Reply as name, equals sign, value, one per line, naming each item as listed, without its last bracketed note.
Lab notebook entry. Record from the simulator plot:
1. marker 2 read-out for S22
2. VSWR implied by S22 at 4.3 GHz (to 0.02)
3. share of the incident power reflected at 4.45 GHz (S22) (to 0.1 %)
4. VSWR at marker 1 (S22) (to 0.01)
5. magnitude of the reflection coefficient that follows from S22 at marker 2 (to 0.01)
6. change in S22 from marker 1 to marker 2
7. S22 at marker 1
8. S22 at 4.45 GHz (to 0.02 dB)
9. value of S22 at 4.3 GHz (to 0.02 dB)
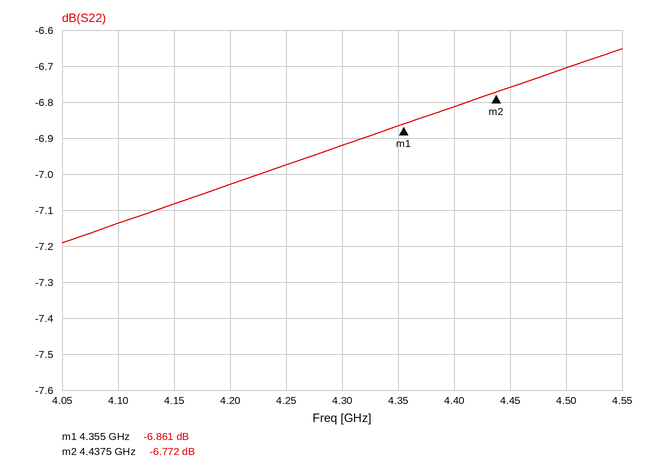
marker 2 read-out for S22 = -6.772 dB
VSWR implied by S22 at 4.3 GHz = 2.64
share of the incident power reflected at 4.45 GHz (S22) = 21.1 %
VSWR at marker 1 (S22) = 2.66
magnitude of the reflection coefficient that follows from S22 at marker 2 = 0.46
change in S22 from marker 1 to marker 2 = 0.089 dB
S22 at marker 1 = -6.861 dB
S22 at 4.45 GHz = -6.76 dB
value of S22 at 4.3 GHz = -6.92 dB
